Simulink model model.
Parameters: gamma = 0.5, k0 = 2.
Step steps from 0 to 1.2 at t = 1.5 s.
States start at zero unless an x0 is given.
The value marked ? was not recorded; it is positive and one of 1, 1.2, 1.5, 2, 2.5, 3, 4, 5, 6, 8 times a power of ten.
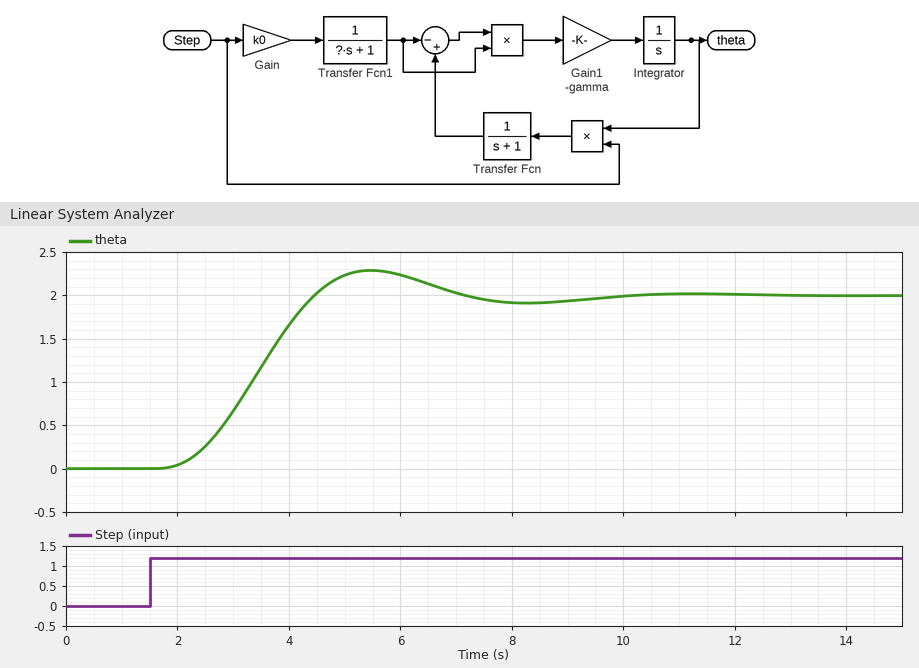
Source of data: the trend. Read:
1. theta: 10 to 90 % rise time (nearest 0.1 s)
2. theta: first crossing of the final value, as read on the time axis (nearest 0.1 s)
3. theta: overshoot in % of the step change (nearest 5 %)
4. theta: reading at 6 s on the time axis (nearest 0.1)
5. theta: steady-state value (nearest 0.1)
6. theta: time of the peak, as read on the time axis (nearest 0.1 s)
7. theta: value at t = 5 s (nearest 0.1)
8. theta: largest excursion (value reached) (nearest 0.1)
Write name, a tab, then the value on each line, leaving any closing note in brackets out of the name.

theta: 10 to 90 % rise time	1.8 s
theta: first crossing of the final value, as read on the time axis	4.5 s
theta: overshoot in % of the step change	15 %
theta: reading at 6 s on the time axis	2.2
theta: steady-state value	2.0
theta: time of the peak, as read on the time axis	5.5 s
theta: value at t = 5 s	2.2
theta: largest excursion (value reached)	2.3
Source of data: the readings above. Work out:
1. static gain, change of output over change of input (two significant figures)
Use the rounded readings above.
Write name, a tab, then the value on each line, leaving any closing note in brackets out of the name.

static gain, change of output over change of input	1.7
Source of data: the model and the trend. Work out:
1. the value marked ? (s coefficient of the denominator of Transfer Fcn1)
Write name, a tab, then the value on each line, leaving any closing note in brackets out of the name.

the value marked ?	1.5
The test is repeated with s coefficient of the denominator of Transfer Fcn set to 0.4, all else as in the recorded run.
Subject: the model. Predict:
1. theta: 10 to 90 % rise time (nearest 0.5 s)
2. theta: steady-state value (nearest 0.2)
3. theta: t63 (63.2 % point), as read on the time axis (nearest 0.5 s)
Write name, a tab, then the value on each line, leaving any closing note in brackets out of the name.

theta: 10 to 90 % rise time	2.5 s
theta: steady-state value	2.0
theta: t63 (63.2 % point), as read on the time axis	4.0 s
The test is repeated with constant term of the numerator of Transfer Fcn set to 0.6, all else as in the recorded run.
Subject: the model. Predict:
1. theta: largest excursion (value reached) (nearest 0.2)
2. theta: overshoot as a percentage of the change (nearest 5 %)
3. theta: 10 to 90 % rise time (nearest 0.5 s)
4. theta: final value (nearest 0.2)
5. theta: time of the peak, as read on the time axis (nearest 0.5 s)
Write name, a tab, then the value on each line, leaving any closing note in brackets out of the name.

theta: largest excursion (value reached)	3.6
theta: overshoot as a percentage of the change	10 %
theta: 10 to 90 % rise time	2.5 s
theta: final value	3.4
theta: time of the peak, as read on the time axis	7.0 s
